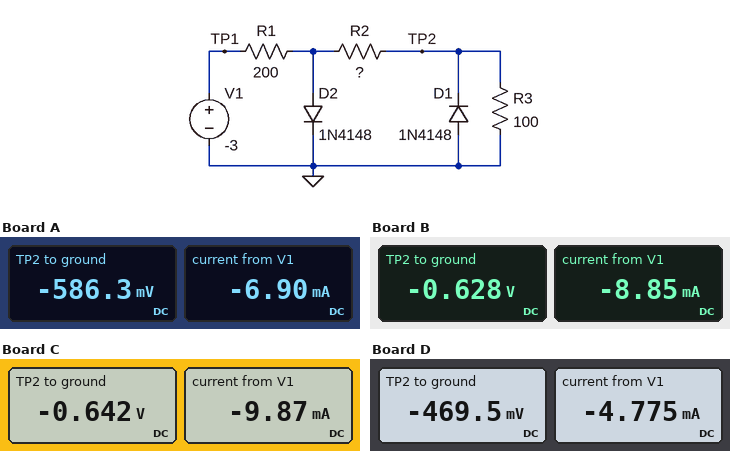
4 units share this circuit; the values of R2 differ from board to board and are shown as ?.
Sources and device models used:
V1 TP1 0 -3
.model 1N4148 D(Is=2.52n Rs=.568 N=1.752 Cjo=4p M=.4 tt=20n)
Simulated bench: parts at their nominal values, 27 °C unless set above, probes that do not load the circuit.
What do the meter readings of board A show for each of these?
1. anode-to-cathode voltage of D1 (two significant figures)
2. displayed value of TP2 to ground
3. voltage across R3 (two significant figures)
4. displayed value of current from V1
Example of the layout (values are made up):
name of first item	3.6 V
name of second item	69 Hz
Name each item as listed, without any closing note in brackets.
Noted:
anode-to-cathode voltage of D1	590 mV
displayed value of TP2 to ground	-586.3 mV
voltage across R3	590 mV
displayed value of current from V1	-6.90 mA
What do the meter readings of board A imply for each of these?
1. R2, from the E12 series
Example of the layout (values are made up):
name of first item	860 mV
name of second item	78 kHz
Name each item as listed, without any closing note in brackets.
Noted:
R2, from the E12 series	150 Ω
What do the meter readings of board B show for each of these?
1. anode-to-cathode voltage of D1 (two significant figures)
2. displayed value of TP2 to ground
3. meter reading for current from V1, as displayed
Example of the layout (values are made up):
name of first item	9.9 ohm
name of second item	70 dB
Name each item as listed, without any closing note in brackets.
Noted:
anode-to-cathode voltage of D1	630 mV
displayed value of TP2 to ground	-0.628 V
meter reading for current from V1, as displayed	-8.85 mA
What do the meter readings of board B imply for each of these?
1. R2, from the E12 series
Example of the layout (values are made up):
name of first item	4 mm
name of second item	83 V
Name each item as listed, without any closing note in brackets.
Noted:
R2, from the E12 series	68 Ω
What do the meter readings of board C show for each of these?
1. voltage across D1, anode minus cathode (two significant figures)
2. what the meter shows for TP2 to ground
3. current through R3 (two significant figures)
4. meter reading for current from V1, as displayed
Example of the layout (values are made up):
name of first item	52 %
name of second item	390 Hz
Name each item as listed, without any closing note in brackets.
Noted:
voltage across D1, anode minus cathode	640 mV
what the meter shows for TP2 to ground	-0.642 V
current through R3	6.4 mA
meter reading for current from V1, as displayed	-9.87 mA
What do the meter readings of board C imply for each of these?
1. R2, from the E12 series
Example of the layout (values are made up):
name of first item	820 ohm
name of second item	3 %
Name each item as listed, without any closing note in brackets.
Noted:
R2, from the E12 series	39 Ω
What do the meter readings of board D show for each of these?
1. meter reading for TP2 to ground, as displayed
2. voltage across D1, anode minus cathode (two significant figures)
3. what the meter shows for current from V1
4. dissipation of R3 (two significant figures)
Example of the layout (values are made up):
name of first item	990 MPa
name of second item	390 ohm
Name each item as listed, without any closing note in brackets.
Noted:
meter reading for TP2 to ground, as displayed	-469.5 mV
voltage across D1, anode minus cathode	470 mV
what the meter shows for current from V1	-4.775 mA
dissipation of R3	2.2 mW
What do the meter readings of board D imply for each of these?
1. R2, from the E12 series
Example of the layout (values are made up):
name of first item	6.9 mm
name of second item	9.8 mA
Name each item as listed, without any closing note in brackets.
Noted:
R2, from the E12 series	330 Ω
